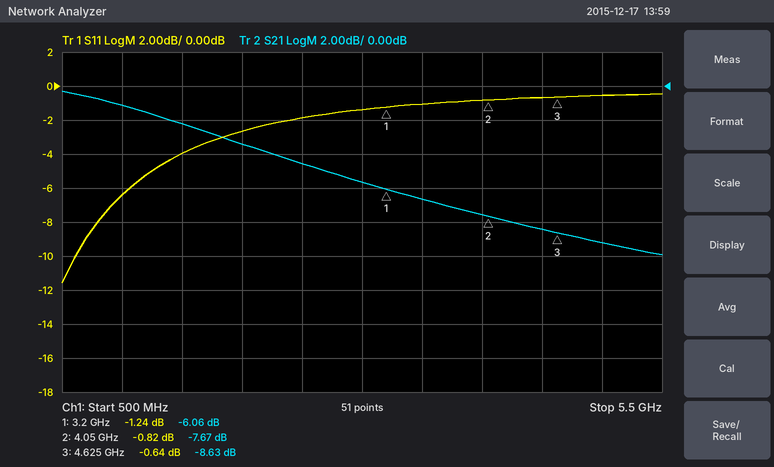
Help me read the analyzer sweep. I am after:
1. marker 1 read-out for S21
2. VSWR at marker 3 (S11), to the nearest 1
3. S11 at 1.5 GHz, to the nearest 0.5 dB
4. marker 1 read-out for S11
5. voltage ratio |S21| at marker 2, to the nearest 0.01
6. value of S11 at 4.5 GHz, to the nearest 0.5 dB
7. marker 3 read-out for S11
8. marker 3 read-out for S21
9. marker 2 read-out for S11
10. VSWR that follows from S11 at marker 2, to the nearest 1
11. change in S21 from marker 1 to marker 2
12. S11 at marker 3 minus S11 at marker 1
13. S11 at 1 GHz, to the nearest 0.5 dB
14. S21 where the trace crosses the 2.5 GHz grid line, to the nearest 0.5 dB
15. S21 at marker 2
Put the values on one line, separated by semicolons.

-6.06 dB; 27; -4.0 dB; -1.24 dB; 0.41; -0.5 dB; -0.64 dB; -8.63 dB; -0.82 dB; 21; -1.61 dB; 0.60 dB; -6.5 dB; -4.5 dB; -7.67 dB
